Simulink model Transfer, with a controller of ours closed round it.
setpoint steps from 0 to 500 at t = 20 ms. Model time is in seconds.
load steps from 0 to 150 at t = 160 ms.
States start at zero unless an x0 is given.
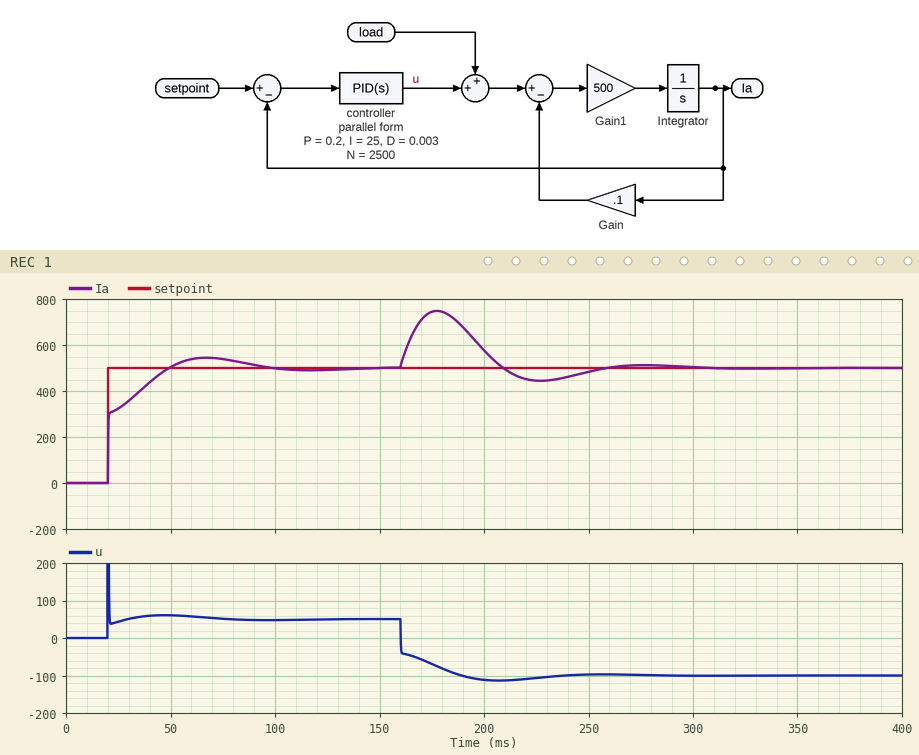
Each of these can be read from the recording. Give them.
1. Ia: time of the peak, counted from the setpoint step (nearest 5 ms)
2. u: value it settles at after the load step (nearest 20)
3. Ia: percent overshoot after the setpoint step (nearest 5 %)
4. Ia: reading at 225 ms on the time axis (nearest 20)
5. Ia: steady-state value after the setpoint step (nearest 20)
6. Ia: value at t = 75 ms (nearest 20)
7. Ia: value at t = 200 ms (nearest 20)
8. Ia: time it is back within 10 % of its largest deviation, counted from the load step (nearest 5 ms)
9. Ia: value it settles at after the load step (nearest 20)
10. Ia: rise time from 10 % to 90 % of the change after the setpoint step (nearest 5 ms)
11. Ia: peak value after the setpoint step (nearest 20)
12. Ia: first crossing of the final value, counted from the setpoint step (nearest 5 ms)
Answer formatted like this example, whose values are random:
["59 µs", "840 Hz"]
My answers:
["45 ms", "-100", "10 %", "440", "500", "540", "580", "85 ms", "500", "20 ms", "540", "30 ms"]
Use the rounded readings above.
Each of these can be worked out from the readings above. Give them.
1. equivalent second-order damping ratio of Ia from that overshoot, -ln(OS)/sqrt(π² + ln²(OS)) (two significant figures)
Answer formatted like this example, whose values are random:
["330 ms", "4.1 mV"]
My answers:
["0.59"]
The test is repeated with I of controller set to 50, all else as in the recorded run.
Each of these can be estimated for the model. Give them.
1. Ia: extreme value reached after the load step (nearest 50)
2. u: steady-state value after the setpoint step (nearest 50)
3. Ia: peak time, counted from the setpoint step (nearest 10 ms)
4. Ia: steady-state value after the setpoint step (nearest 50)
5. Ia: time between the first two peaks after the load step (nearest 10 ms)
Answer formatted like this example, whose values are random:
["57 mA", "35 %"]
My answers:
["700", "50", "30 ms", "500", "70 ms"]
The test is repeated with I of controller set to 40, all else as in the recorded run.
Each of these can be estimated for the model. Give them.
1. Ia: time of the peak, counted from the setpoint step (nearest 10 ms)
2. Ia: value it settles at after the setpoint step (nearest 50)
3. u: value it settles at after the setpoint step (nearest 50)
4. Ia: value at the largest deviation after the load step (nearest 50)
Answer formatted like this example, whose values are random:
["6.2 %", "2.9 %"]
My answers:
["40 ms", "500", "50", "700"]
